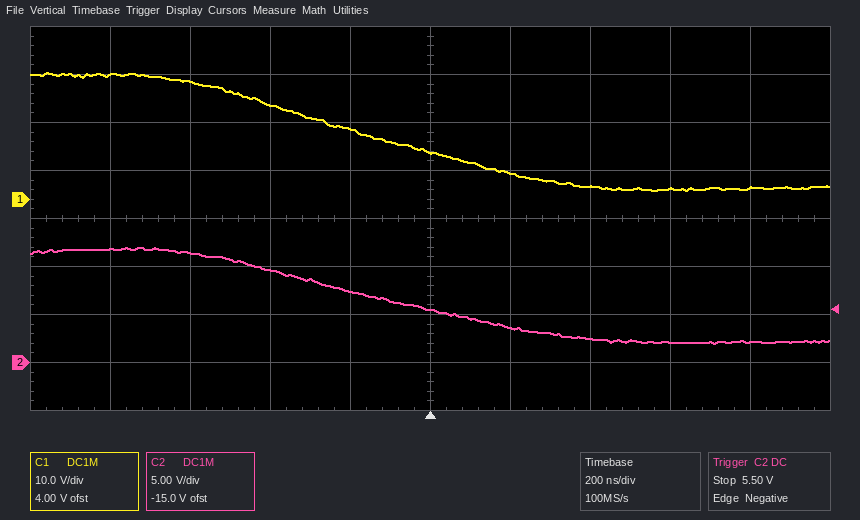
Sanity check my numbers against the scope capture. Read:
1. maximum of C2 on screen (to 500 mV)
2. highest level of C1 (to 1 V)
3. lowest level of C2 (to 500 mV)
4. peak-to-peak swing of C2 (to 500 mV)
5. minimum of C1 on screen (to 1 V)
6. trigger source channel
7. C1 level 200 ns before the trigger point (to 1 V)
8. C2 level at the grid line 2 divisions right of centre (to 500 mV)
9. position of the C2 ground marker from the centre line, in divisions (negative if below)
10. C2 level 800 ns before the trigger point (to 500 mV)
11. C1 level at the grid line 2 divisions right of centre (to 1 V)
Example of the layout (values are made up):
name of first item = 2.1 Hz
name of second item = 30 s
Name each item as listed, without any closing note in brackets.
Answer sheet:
maximum of C2 on screen = 12.0 V
highest level of C1 = 26 V
lowest level of C2 = 2.0 V
peak-to-peak swing of C2 = 10.0 V
minimum of C1 on screen = 2 V
trigger source channel = C2
C1 level 200 ns before the trigger point = 15 V
C2 level at the grid line 2 divisions right of centre = 2.5 V
position of the C2 ground marker from the centre line, in divisions = -3.0 div
C2 level 800 ns before the trigger point = 12.0 V
C1 level at the grid line 2 divisions right of centre = 3 V
